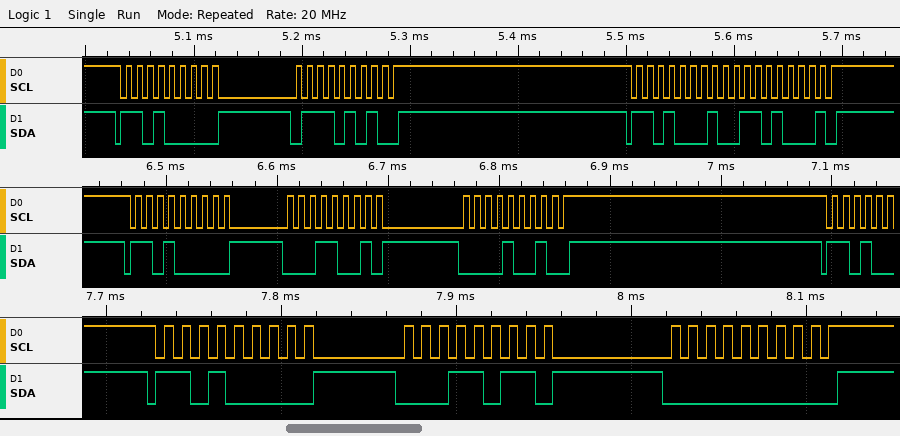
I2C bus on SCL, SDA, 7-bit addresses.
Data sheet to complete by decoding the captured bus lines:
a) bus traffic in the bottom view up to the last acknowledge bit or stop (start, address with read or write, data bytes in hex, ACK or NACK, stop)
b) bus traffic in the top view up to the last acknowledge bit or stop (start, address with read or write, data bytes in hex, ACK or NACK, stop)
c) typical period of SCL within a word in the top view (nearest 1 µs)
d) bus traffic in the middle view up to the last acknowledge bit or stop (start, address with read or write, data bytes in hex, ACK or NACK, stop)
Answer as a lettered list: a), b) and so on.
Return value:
a) start, address 68 write ACK, 1B ACK, 00 ACK, stop
b) start, address 68 write ACK, 75 ACK, stop, start, address 68 read ACK, 68 NACK, stop
c) 10 µs
d) start, address 68 write ACK, 19 ACK, 09 ACK, stop
